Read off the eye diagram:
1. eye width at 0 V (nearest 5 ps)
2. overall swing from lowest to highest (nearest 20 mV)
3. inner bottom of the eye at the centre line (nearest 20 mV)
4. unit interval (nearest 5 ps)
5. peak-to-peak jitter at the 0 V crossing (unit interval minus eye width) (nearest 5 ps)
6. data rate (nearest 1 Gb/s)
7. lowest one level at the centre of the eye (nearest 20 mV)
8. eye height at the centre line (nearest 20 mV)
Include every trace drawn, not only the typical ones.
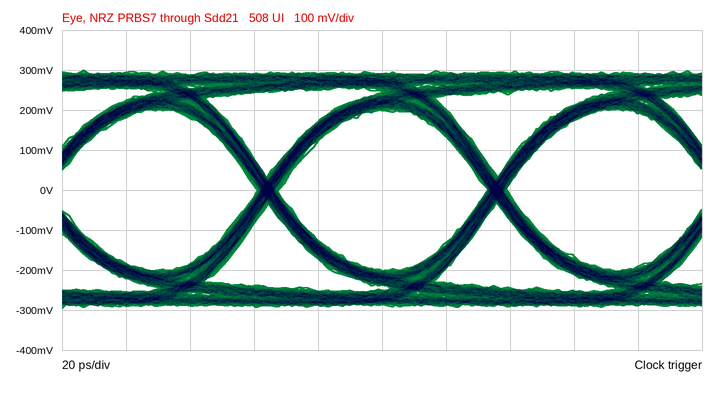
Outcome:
65 ps
600 mV
-200 mV
70 ps
5 ps
14 Gb/s
200 mV
400 mV
